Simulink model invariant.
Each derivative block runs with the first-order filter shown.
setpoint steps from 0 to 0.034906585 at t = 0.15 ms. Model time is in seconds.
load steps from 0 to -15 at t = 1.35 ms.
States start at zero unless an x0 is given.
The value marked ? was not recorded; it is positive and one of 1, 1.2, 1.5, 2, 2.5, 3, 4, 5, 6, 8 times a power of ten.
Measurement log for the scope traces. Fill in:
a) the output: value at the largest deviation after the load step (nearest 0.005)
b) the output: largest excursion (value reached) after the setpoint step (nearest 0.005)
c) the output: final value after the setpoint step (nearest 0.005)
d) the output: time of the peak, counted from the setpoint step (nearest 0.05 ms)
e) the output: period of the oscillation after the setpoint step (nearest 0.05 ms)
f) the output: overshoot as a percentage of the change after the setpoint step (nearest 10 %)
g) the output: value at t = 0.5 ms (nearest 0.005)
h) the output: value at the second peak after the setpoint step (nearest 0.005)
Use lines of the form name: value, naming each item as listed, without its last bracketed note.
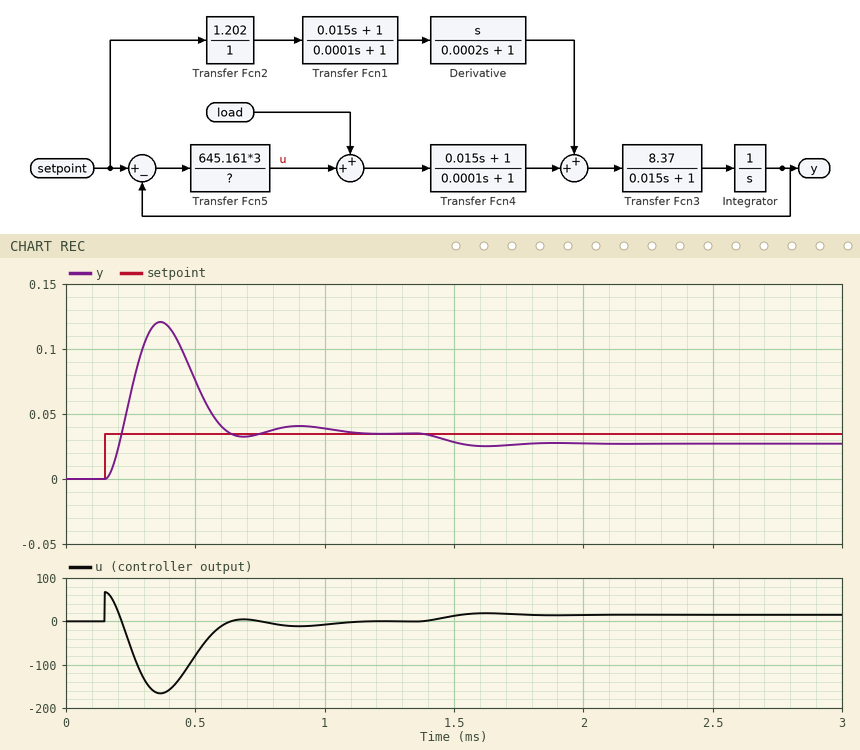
the output: value at the largest deviation after the load step: 0.025
the output: largest excursion (value reached) after the setpoint step: 0.120
the output: final value after the setpoint step: 0.035
the output: time of the peak, counted from the setpoint step: 0.20 ms
the output: period of the oscillation after the setpoint step: 0.55 ms
the output: overshoot as a percentage of the change after the setpoint step: 250 %
the output: value at t = 0.5 ms: 0.075
the output: value at the second peak after the setpoint step: 0.040
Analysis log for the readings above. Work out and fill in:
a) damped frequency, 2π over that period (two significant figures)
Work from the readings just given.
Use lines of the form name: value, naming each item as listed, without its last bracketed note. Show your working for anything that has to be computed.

damped frequency, 2π over that period: 2π / 0.55 = 11 rad/ms
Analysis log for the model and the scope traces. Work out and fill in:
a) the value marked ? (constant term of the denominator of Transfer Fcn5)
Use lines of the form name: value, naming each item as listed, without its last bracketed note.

the value marked ?: 1
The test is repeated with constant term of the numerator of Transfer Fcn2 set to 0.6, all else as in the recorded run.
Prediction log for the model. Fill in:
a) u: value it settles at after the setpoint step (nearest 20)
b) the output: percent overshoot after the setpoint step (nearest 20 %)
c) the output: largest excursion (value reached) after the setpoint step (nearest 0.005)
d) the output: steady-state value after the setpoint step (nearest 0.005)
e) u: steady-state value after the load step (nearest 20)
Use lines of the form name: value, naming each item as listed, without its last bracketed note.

u: value it settles at after the setpoint step: 0
the output: percent overshoot after the setpoint step: 140 %
the output: largest excursion (value reached) after the setpoint step: 0.080
the output: steady-state value after the setpoint step: 0.035
u: steady-state value after the load step: 20
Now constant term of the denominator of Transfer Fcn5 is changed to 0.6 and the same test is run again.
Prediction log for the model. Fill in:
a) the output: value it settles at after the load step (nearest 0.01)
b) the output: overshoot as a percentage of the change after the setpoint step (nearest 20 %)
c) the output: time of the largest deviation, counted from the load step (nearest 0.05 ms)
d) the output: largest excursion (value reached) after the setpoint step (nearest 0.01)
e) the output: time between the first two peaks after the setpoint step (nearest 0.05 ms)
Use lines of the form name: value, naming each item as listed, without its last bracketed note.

the output: value it settles at after the load step: 0.03
the output: overshoot as a percentage of the change after the setpoint step: 200 %
the output: time of the largest deviation, counted from the load step: 0.20 ms
the output: largest excursion (value reached) after the setpoint step: 0.10
the output: time between the first two peaks after the setpoint step: 0.40 ms
